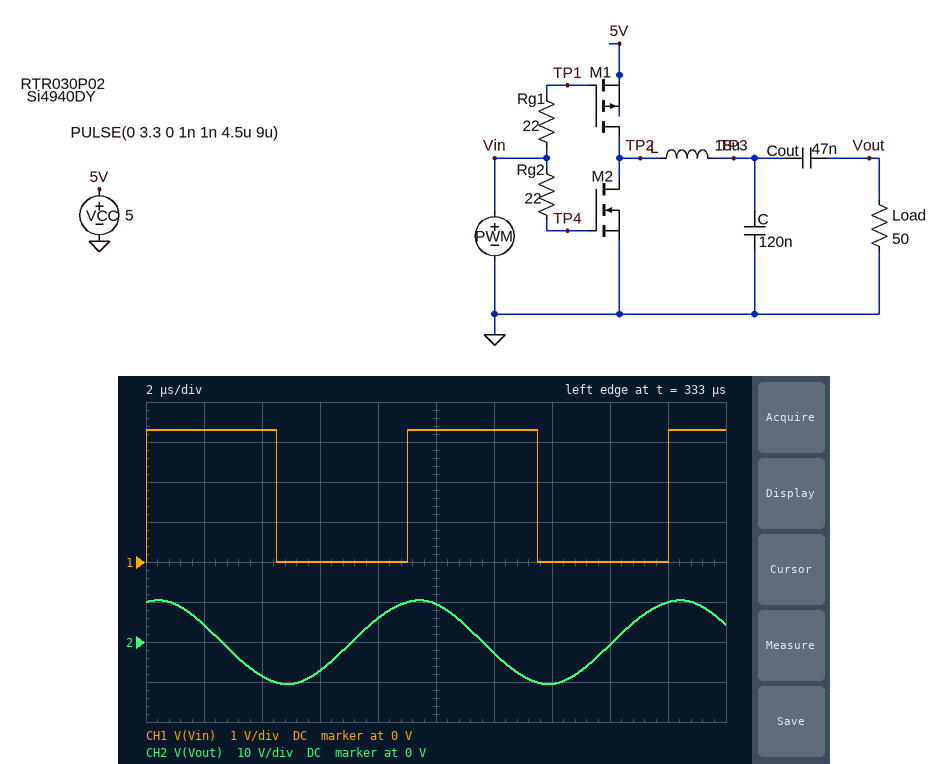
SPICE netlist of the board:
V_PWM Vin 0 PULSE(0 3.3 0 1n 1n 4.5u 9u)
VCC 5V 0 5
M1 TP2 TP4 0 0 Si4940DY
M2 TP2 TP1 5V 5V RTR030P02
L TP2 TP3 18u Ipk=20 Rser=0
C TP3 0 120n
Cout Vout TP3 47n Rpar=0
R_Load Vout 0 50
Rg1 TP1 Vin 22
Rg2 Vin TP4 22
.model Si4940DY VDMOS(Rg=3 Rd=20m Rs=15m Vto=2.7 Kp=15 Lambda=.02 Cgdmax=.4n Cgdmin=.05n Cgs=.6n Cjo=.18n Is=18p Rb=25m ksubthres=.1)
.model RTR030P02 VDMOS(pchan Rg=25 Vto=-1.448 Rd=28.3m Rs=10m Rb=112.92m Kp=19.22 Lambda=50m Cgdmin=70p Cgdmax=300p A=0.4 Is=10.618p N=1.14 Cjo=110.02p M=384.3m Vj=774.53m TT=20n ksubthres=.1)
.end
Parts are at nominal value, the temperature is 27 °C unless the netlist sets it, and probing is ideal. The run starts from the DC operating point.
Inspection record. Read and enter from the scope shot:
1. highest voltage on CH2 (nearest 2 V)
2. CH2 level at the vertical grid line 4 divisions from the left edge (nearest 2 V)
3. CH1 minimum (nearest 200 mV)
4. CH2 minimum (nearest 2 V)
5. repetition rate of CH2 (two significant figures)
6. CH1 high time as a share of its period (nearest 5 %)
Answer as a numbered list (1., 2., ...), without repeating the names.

1. 10 V
2. 6 V
3. 0 V
4. -10 V
5. 110 kHz
6. 50 %
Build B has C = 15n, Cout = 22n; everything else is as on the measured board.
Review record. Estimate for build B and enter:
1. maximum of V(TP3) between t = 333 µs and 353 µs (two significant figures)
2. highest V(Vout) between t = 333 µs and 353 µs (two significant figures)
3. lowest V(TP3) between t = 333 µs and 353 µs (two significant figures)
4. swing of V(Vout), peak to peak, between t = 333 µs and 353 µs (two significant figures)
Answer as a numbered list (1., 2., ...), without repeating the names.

1. 7.5 V
2. 3.6 V
3. -2.5 V
4. 7.4 V
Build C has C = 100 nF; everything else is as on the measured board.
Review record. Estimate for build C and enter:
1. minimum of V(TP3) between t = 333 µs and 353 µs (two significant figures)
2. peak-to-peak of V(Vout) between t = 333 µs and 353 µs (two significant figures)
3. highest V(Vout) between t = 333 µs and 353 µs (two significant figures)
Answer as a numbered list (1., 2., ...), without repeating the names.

1. -13 V
2. 27 V
3. 13 V
